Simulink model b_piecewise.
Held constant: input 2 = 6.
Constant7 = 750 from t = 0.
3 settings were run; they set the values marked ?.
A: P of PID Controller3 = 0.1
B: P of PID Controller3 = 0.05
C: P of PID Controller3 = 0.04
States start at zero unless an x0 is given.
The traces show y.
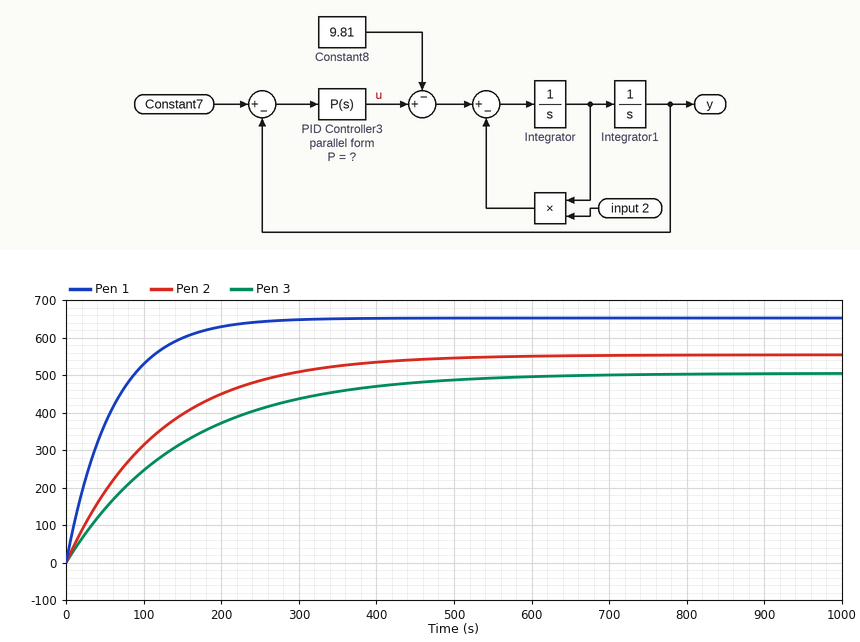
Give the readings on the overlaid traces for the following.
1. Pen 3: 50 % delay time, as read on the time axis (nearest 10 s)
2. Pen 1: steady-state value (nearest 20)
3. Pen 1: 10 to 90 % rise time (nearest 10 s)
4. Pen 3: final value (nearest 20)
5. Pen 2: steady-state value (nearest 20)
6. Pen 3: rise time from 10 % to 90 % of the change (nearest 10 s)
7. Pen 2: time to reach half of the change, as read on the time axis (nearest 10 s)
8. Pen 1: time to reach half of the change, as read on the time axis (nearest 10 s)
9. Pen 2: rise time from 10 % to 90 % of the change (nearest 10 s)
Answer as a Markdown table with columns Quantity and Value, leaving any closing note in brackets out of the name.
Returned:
| Quantity | Value |
|---|---|
| Pen 3: 50 % delay time, as read on the time axis | 100 s |
| Pen 1: steady-state value | 660 |
| Pen 1: 10 to 90 % rise time | 130 s |
| Pen 3: final value | 500 |
| Pen 2: steady-state value | 560 |
| Pen 3: rise time from 10 % to 90 % of the change | 330 s |
| Pen 2: time to reach half of the change, as read on the time axis | 80 s |
| Pen 1: time to reach half of the change, as read on the time axis | 40 s |
| Pen 2: rise time from 10 % to 90 % of the change | 260 s |
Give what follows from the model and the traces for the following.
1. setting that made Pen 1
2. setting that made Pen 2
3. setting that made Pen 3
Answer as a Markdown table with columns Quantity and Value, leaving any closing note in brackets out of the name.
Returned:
| Quantity | Value |
|---|---|
| setting that made Pen 1 | A |
| setting that made Pen 2 | B |
| setting that made Pen 3 | C |
